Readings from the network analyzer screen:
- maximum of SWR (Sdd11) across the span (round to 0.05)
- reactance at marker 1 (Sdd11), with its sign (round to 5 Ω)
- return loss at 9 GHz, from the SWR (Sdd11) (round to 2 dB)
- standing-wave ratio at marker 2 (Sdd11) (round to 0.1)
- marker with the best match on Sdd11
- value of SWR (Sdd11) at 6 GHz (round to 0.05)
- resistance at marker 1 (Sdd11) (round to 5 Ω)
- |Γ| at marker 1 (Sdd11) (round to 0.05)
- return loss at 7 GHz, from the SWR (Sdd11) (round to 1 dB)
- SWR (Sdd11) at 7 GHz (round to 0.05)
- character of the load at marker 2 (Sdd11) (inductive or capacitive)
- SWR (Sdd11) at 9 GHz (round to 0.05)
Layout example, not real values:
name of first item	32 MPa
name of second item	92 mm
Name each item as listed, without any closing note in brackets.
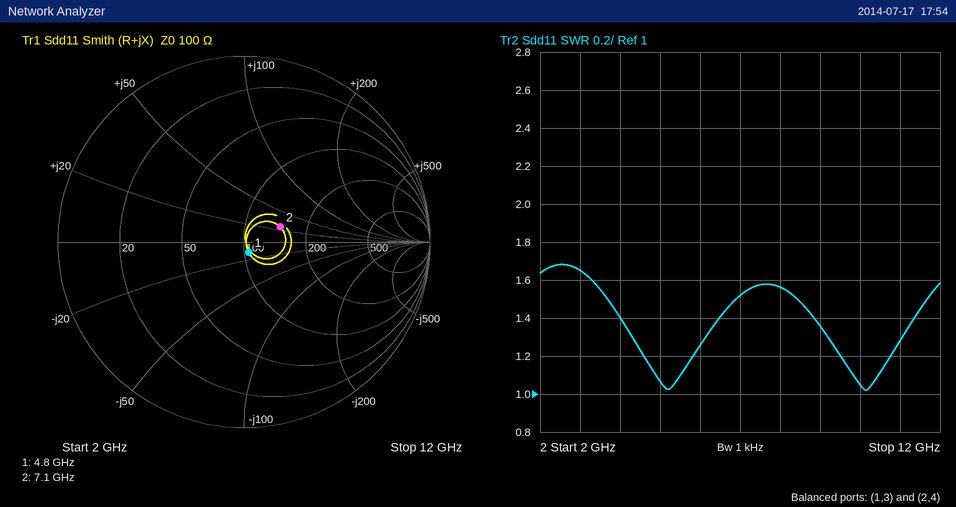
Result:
maximum of SWR (Sdd11) across the span	1.70
reactance at marker 1 (Sdd11), with its sign	-10 Ω
return loss at 9 GHz, from the SWR (Sdd11)	16 dB
standing-wave ratio at marker 2 (Sdd11)	1.5
marker with the best match on Sdd11	marker 1
value of SWR (Sdd11) at 6 GHz	1.25
resistance at marker 1 (Sdd11)	105 Ω
|Γ| at marker 1 (Sdd11)	0.05
return loss at 7 GHz, from the SWR (Sdd11)	14 dB
SWR (Sdd11) at 7 GHz	1.50
character of the load at marker 2 (Sdd11)	inductive
SWR (Sdd11) at 9 GHz	1.35
